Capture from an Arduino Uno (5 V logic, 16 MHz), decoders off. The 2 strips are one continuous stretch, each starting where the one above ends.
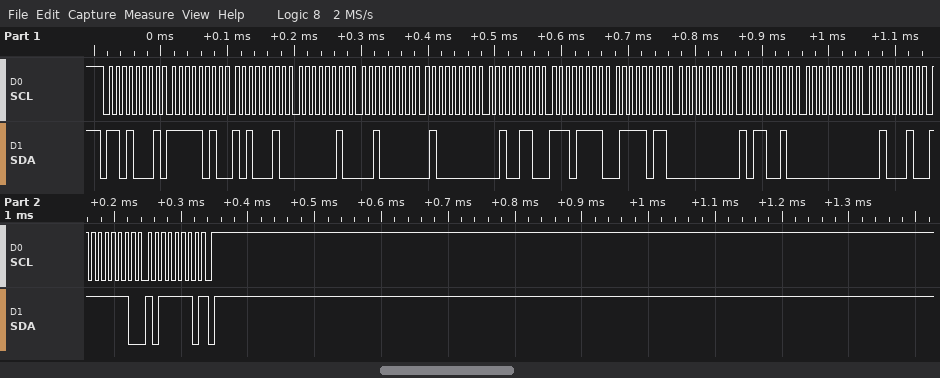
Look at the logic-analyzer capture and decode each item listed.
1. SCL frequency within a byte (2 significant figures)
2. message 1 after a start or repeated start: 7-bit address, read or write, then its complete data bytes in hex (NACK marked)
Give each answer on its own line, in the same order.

100 kHz
0x68 read: FA A2 02 20 40 26 EF 7B 00 B2 00 22 FE BE NACK
